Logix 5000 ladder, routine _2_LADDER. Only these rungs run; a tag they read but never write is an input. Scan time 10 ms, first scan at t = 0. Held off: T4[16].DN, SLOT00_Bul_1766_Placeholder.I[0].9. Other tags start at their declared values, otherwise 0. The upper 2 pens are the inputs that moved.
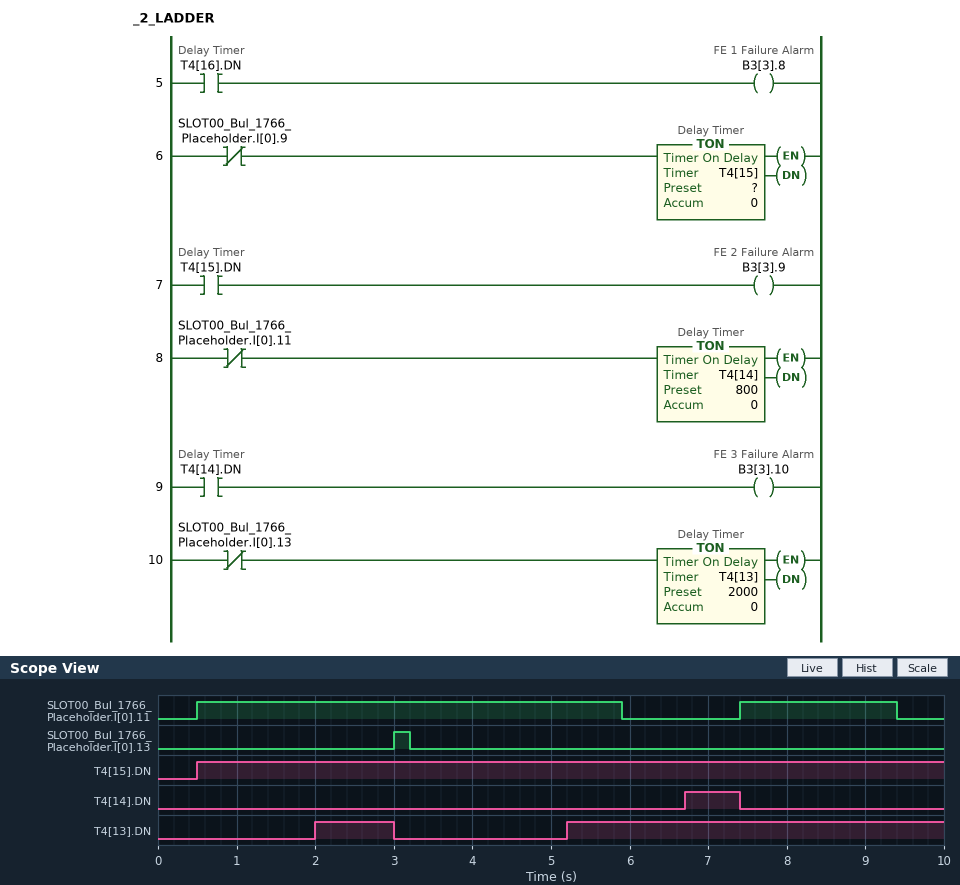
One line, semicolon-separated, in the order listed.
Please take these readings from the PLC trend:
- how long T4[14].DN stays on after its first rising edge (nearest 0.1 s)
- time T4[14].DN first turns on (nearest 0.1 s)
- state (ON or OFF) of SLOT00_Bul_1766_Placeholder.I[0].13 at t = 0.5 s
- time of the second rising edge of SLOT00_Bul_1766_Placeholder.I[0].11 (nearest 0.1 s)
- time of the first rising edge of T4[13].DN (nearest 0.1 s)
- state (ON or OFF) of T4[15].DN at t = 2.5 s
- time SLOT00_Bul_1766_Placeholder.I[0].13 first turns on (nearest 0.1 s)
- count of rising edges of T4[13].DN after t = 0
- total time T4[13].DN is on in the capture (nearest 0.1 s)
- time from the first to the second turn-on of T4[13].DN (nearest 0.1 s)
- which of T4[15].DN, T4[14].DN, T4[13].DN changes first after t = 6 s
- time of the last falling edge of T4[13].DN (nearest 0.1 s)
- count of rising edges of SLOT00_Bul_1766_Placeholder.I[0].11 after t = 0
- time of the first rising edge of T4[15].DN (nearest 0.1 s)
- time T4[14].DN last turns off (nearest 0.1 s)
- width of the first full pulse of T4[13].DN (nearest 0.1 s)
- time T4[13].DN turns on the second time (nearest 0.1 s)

0.7 s; 6.7 s; OFF; 7.4 s; 2.0 s; ON; 3.0 s; 2; 5.8 s; 3.2 s; T4[14].DN; 3.0 s; 2; 0.5 s; 7.4 s; 1.0 s; 5.2 s
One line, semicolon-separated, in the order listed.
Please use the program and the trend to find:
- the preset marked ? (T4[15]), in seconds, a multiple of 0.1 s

0.5 s
